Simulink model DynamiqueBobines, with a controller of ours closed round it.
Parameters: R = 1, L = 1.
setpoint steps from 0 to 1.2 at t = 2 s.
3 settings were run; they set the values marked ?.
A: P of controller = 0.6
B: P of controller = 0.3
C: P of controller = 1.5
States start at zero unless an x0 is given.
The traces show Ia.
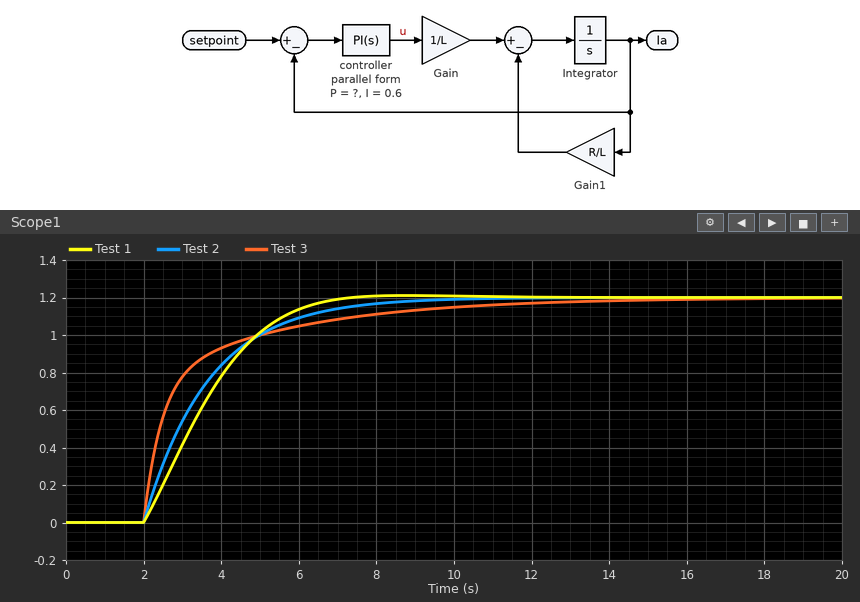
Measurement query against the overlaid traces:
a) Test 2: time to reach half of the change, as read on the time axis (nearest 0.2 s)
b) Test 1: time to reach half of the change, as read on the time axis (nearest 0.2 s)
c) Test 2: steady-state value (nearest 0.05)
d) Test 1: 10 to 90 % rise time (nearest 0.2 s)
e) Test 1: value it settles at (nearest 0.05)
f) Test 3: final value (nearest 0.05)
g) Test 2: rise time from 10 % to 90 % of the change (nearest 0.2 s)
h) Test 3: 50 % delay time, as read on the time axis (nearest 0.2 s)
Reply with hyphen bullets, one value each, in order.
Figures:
- 3.2 s
- 3.4 s
- 1.20
- 3.2 s
- 1.20
- 1.20
- 3.6 s
- 2.6 s
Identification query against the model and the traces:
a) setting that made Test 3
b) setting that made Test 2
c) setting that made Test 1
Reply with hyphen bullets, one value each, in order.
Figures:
- C
- A
- B
